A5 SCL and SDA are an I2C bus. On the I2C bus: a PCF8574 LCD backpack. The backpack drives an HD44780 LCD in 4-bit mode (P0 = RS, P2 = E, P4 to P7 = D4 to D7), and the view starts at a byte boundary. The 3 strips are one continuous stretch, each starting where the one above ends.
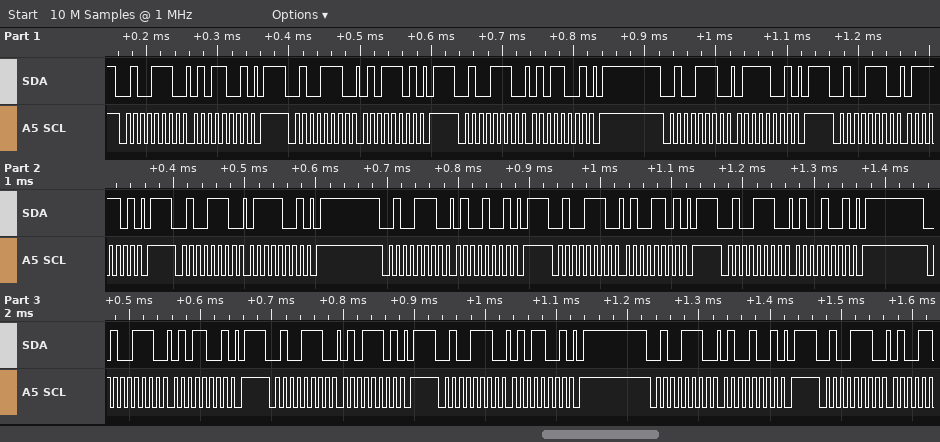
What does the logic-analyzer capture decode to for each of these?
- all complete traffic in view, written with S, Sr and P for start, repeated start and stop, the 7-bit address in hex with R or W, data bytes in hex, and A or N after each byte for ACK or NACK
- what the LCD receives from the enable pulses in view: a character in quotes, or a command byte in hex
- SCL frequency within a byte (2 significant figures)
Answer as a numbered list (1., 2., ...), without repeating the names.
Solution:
1. S 27W A 59 A P S 27W A 5D A P S 27W A 59 A P S 27W A 79 A P S 27W A 7D A P S 27W A 79 A P S 27W A 49 A P S 27W A 4D A P S 27W A 49 A P S 27W A 59 A P S 27W A 5D A P S 27W A 59 A P S 27W A 49 A P S 27W A
2. 'W' 'E'
3. 100 kHz
